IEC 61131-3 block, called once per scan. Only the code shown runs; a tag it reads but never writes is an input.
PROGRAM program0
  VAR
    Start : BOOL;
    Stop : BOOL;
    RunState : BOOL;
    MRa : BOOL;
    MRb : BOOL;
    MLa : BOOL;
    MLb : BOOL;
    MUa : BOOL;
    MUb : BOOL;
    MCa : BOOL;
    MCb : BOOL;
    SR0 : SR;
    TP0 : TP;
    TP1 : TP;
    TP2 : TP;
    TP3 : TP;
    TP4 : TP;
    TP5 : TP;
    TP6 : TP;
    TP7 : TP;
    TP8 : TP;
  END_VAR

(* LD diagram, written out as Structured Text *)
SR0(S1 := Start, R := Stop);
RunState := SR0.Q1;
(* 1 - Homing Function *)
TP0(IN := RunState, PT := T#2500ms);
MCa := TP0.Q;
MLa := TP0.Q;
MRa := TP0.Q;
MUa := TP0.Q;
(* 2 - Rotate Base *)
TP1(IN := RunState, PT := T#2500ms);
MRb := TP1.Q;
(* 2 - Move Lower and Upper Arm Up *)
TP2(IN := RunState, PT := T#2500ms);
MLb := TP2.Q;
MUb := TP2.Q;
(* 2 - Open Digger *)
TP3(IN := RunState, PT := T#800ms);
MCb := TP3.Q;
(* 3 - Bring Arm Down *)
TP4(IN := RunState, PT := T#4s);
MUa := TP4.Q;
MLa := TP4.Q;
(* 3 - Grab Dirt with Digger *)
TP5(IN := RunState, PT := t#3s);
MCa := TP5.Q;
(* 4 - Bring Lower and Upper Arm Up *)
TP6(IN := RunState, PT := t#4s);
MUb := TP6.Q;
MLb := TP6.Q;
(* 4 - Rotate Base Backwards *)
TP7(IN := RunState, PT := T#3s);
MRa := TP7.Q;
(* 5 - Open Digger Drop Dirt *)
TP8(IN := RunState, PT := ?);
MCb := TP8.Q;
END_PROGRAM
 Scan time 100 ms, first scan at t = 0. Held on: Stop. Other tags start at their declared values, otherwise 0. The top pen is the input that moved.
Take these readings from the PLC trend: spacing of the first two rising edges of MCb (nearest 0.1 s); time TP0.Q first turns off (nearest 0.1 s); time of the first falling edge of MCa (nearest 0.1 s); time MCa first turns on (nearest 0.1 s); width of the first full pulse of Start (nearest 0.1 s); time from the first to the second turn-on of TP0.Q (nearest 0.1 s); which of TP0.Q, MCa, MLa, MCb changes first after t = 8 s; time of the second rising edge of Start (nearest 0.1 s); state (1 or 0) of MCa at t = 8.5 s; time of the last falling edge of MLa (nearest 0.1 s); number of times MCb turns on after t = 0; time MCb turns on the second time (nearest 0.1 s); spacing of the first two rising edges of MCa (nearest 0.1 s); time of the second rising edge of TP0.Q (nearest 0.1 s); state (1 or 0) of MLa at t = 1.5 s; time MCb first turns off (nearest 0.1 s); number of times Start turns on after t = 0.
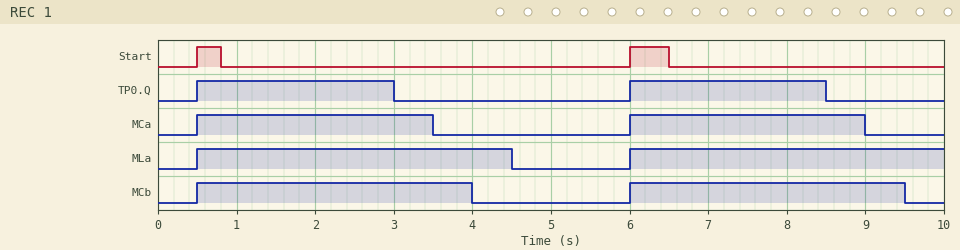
5.5 s
3.0 s
3.5 s
0.5 s
0.3 s
5.5 s
TP0.Q
6.0 s
1
4.5 s
2
6.0 s
5.5 s
6.0 s
1
4.0 s
2
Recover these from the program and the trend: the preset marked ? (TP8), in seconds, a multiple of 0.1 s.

3.5 s
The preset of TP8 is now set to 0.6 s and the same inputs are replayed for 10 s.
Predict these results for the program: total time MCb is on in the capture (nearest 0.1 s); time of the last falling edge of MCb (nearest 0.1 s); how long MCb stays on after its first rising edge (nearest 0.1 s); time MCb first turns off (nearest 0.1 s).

1.2 s
6.6 s
0.6 s
1.1 s
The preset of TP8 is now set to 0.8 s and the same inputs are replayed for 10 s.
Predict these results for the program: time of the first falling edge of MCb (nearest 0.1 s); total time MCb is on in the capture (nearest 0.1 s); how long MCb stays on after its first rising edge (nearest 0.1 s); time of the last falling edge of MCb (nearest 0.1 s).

1.3 s
1.6 s
0.8 s
6.8 s
